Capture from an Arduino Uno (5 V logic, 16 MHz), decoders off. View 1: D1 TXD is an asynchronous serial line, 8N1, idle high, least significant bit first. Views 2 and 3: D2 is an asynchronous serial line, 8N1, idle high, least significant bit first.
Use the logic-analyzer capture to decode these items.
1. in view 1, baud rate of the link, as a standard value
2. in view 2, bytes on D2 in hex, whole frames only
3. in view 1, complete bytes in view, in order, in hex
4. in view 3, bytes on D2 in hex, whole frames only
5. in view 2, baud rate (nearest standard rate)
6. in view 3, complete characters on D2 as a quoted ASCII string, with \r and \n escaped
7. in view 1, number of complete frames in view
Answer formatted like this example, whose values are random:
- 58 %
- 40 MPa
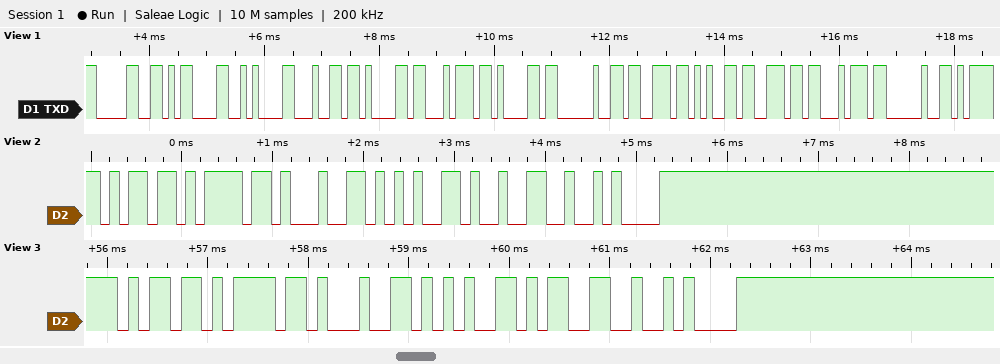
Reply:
- 9600 baud
- 0x6D 0x6F 0x64 0x65 0x32 0x0A
- 30 0D 0A 64 61 74 61 20 73 65 6E 74 20
- 6D 6F 64 65 33 0A
- 9600 baud
- "mode3\n"
- 13
